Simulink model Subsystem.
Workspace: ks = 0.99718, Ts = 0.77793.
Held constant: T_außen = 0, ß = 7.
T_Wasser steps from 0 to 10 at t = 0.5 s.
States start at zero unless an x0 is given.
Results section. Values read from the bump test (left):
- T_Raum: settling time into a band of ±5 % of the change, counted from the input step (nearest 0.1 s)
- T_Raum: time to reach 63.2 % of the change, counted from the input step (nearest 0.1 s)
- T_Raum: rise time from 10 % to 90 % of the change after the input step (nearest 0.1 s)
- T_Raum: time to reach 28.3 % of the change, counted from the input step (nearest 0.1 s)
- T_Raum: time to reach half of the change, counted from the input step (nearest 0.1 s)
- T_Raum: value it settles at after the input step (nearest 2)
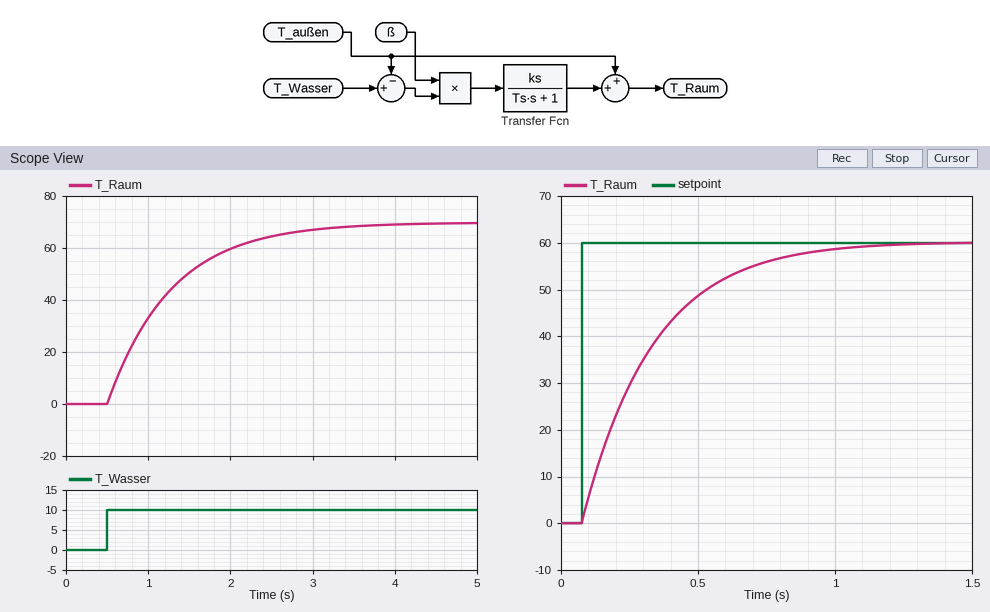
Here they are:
2.3 s
0.8 s
1.7 s
0.3 s
0.5 s
70
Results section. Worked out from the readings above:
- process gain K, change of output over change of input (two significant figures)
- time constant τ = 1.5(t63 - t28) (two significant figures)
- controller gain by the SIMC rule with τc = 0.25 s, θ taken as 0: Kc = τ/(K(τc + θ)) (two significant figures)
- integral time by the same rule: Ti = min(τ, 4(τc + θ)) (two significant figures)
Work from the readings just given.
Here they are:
7.0
0.75 s
0.43
0.75 s
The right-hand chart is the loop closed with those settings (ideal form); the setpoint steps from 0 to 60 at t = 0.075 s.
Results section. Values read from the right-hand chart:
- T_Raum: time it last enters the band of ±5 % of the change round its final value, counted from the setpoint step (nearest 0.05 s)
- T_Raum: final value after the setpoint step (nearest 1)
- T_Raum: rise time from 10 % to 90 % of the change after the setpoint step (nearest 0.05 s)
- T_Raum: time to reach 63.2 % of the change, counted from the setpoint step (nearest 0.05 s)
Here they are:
0.75 s
60
0.55 s
0.25 s
